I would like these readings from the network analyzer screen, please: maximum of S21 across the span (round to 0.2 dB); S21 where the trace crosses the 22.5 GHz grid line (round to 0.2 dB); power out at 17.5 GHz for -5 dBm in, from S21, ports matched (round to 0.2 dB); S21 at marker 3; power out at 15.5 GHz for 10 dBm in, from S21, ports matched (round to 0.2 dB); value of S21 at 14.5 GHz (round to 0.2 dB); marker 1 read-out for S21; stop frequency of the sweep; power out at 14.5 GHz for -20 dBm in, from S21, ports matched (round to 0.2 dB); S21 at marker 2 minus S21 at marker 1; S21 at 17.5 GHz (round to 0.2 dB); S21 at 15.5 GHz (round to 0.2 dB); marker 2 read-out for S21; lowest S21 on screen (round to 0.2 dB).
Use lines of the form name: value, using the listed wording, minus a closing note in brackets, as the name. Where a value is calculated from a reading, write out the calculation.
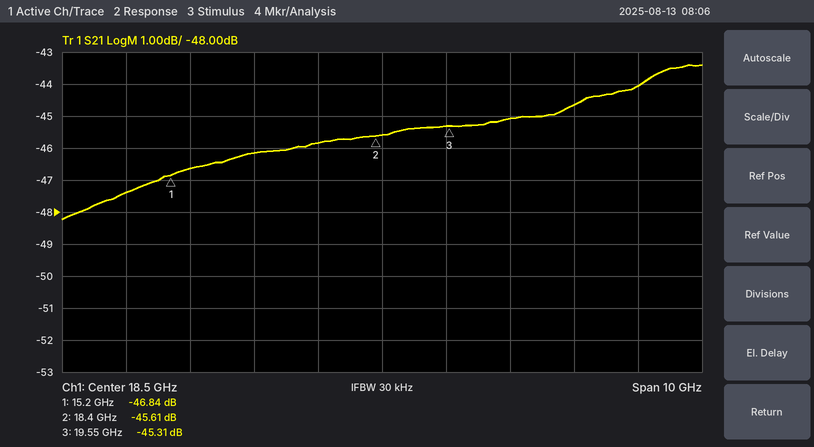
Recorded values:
maximum of S21 across the span: -43.4 dB
S21 where the trace crosses the 22.5 GHz grid line: -44.0 dB
power out at 17.5 GHz for -5 dBm in, from S21, ports matched: -5 dBm + (-45.8 dB) = -50.8 dBm
S21 at marker 3: -45.31 dB
power out at 15.5 GHz for 10 dBm in, from S21, ports matched: 10 dBm + (-46.6 dB) = -36.6 dBm
value of S21 at 14.5 GHz: -47.4 dB
marker 1 read-out for S21: -46.84 dB
stop frequency of the sweep: 23.5 GHz
power out at 14.5 GHz for -20 dBm in, from S21, ports matched: -20 dBm + (-47.4 dB) = -67.4 dBm
S21 at marker 2 minus S21 at marker 1: -45.61 − (-46.84) = 1.23 dB
S21 at 17.5 GHz: -45.8 dB
S21 at 15.5 GHz: -46.6 dB
marker 2 read-out for S21: -45.61 dB
lowest S21 on screen: -48.2 dB
